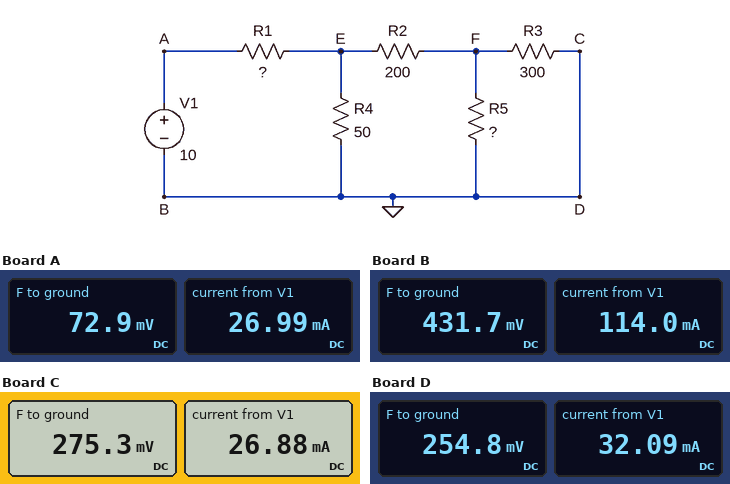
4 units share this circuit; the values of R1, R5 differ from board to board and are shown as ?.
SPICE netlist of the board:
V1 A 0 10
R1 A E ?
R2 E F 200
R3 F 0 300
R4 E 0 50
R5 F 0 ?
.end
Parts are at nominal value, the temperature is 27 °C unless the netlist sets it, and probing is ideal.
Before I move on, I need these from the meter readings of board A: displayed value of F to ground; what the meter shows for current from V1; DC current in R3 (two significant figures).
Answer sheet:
72.9 mV
26.99 mA
240 µA
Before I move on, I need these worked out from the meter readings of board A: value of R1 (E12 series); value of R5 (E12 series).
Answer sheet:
330 Ω
15 Ω
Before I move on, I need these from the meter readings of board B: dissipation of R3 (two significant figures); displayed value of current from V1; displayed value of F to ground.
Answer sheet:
620 µW
114.0 mA
431.7 mV
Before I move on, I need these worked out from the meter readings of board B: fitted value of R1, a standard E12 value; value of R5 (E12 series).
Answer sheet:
47 Ω
22 Ω
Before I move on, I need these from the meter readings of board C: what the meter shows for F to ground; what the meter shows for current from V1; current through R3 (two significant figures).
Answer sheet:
275.3 mV
26.88 mA
920 µA
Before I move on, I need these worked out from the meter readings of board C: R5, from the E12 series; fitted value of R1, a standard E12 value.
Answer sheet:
82 Ω
330 Ω
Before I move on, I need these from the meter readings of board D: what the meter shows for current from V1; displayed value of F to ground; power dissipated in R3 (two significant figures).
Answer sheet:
32.09 mA
254.8 mV
220 µW
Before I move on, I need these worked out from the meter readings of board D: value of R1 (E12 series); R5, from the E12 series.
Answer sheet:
270 Ω
56 Ω
